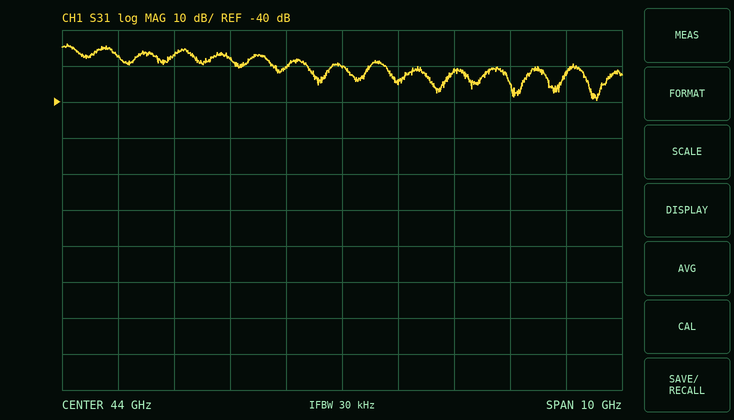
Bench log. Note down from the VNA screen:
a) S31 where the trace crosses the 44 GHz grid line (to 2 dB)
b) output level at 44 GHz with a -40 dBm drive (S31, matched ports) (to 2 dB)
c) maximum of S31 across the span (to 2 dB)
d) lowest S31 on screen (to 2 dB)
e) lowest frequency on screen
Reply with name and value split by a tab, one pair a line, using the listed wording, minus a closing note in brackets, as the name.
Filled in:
S31 where the trace crosses the 44 GHz grid line	-30 dB
output level at 44 GHz with a -40 dBm drive (S31, matched ports)	-70 dBm
maximum of S31 across the span	-24 dB
lowest S31 on screen	-40 dB
lowest frequency on screen	39 GHz
